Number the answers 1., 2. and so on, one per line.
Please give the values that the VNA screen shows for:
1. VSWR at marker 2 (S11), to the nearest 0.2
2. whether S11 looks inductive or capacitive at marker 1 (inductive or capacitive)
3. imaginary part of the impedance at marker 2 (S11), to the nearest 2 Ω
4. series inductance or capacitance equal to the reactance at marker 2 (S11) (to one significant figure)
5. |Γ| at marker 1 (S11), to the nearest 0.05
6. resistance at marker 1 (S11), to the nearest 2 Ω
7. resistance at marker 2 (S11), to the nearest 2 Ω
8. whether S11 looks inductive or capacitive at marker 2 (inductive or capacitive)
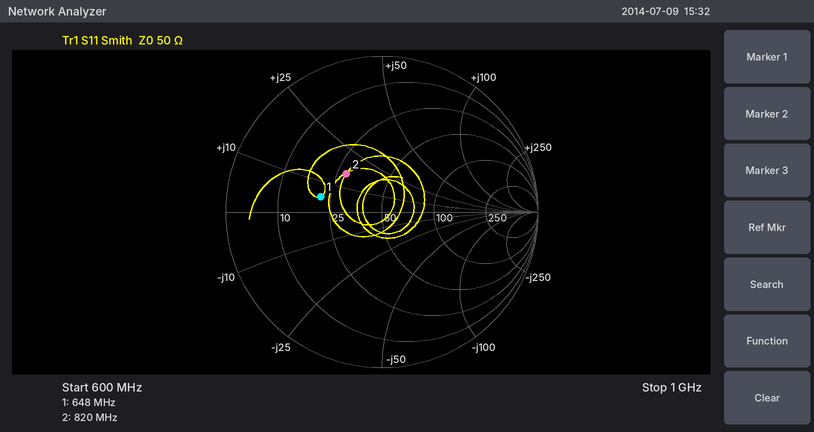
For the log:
1. 2.0
2. inductive
3. +16 Ω
4. 3 nH
5. 0.40
6. 22 Ω
7. 28 Ω
8. inductive
